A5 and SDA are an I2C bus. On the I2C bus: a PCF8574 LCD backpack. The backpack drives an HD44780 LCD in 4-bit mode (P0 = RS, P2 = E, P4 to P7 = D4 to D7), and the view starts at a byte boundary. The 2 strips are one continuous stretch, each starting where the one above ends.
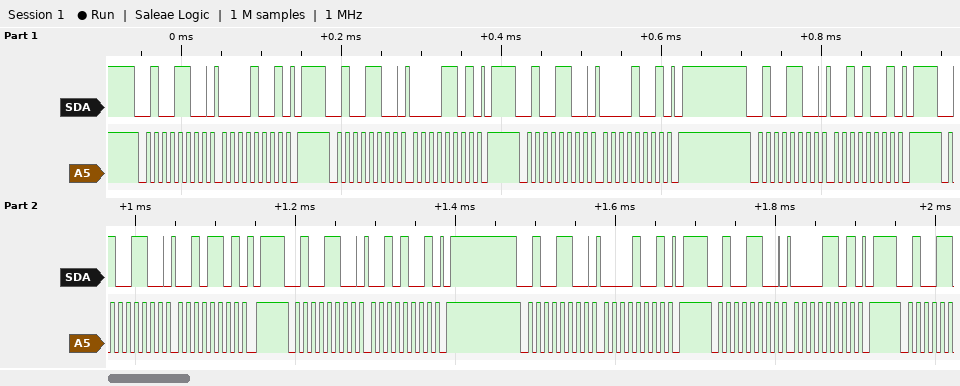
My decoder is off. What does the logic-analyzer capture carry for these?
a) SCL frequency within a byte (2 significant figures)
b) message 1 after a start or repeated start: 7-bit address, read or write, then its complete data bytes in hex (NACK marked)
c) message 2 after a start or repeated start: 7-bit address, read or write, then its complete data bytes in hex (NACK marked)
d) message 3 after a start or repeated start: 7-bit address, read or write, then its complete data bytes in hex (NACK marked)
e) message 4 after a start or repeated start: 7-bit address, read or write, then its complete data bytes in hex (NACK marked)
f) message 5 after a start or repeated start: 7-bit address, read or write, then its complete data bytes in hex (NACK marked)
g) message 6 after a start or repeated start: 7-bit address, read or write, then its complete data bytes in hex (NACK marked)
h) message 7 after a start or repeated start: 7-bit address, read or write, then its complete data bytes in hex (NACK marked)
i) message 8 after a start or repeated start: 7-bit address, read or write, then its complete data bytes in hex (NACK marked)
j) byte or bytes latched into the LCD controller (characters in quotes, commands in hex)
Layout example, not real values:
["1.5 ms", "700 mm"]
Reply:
["100 kHz", "0x26 write: 09", "0x26 write: 0D", "0x26 write: 09", "0x26 write: 29", "0x26 write: 2D", "0x26 write: 29", "0x26 write: 09", "0x26 write: 0D", "data 0x02"]
